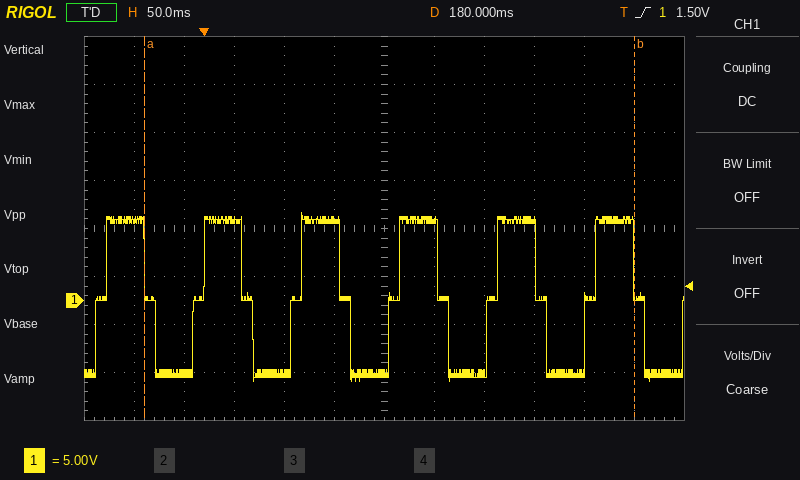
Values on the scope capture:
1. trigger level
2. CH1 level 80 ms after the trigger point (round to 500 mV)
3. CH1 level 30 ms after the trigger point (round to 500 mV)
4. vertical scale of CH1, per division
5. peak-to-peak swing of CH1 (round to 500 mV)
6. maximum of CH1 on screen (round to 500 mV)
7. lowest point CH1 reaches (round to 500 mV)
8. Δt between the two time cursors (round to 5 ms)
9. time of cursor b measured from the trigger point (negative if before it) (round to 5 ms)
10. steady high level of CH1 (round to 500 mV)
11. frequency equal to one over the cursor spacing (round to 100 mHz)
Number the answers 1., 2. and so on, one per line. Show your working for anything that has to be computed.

1. 1.50 V
2. -7.5 V
3. 8.5 V
4. 5 V
5. 9.0 V − (-8.5 V) = 17.5 V
6. 9.0 V
7. -8.5 V
8. 490 ms
9. +430 ms
10. 8.5 V
11. 1 / 490 ms ≈ 2.0 Hz
